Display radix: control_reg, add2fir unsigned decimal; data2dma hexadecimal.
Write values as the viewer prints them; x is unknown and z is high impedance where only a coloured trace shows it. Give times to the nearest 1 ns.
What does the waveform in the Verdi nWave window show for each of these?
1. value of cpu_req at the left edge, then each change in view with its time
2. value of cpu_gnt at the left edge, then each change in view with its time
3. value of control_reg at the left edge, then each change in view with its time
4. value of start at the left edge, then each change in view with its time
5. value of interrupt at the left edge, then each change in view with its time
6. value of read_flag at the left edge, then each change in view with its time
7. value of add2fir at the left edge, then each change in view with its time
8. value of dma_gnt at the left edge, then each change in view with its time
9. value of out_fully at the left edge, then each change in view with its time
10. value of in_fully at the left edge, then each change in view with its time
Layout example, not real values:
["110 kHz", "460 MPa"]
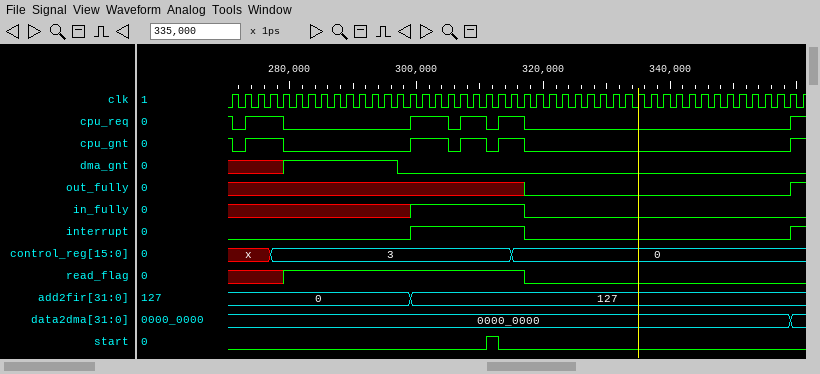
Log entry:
["1, 0 at 271 ns, 1 at 273 ns, 0 at 279 ns, 1 at 299 ns, 0 at 305 ns, 1 at 307 ns, 0 at 311 ns, 1 at 313 ns, 0 at 317 ns, 1 at 359 ns", "1, 0 at 271 ns, 1 at 273 ns, 0 at 279 ns, 1 at 299 ns, 0 at 305 ns, 1 at 307 ns, 0 at 311 ns, 1 at 313 ns, 0 at 317 ns, 1 at 359 ns", "x, 3 at 277 ns, 0 at 315 ns", "0, 1 at 311 ns, 0 at 313 ns", "0, 1 at 299 ns, 0 at 317 ns, 1 at 359 ns", "x, 1 at 279 ns, 0 at 317 ns", "0, 127 at 299 ns", "x, 1 at 279 ns, 0 at 297 ns", "x, 0 at 317 ns, 1 at 359 ns", "x, 1 at 299 ns, 0 at 317 ns"]
